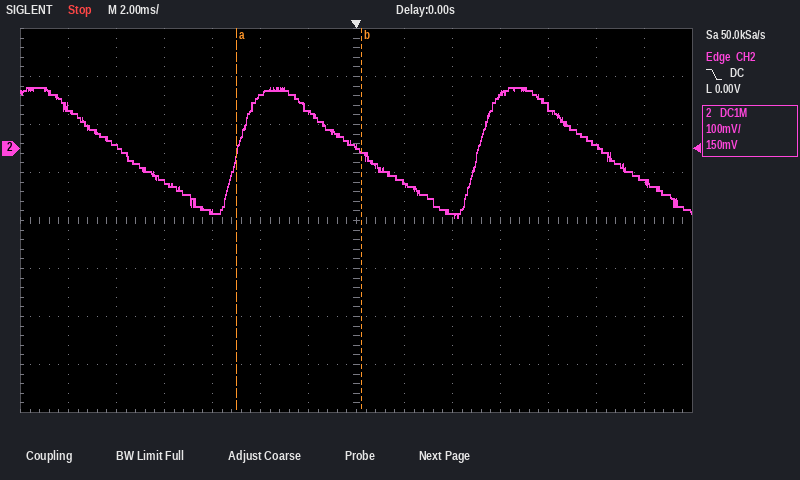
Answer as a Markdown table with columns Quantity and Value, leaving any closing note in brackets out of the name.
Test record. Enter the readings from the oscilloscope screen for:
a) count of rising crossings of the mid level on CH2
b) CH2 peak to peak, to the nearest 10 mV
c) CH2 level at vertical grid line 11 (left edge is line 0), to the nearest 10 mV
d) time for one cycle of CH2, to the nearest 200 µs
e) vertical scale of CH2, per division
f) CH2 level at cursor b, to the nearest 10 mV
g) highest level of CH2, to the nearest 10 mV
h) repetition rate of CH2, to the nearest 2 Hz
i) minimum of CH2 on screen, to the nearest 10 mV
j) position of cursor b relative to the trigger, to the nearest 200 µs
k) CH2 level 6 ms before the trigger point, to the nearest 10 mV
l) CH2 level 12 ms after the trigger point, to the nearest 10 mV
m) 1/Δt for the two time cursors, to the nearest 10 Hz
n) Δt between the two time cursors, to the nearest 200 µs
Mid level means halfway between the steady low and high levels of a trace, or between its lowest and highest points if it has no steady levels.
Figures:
| Quantity | Value |
|---|---|
| count of rising crossings of the mid level on CH2 | 2 |
| CH2 peak to peak, to the nearest 10 mV | 270 mV |
| CH2 level at vertical grid line 11 (left edge is line 0), to the nearest 10 mV | 90 mV |
| time for one cycle of CH2, to the nearest 200 µs | 10.0 ms |
| vertical scale of CH2, per division | 100 mV |
| CH2 level at cursor b, to the nearest 10 mV | -10 mV |
| highest level of CH2, to the nearest 10 mV | 130 mV |
| repetition rate of CH2, to the nearest 2 Hz | 100 Hz |
| minimum of CH2 on screen, to the nearest 10 mV | -140 mV |
| position of cursor b relative to the trigger, to the nearest 200 µs | +200 µs |
| CH2 level 6 ms before the trigger point, to the nearest 10 mV | -130 mV |
| CH2 level 12 ms after the trigger point, to the nearest 10 mV | -70 mV |
| 1/Δt for the two time cursors, to the nearest 10 Hz | 190 Hz |
| Δt between the two time cursors, to the nearest 200 µs | 5.2 ms |
